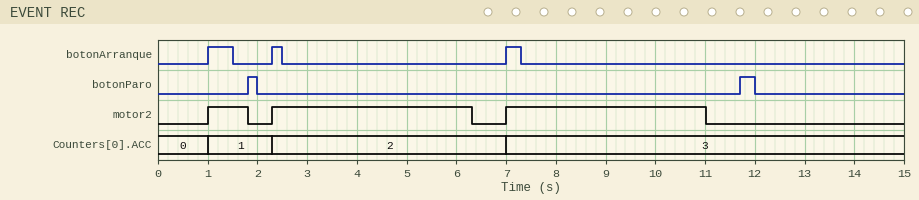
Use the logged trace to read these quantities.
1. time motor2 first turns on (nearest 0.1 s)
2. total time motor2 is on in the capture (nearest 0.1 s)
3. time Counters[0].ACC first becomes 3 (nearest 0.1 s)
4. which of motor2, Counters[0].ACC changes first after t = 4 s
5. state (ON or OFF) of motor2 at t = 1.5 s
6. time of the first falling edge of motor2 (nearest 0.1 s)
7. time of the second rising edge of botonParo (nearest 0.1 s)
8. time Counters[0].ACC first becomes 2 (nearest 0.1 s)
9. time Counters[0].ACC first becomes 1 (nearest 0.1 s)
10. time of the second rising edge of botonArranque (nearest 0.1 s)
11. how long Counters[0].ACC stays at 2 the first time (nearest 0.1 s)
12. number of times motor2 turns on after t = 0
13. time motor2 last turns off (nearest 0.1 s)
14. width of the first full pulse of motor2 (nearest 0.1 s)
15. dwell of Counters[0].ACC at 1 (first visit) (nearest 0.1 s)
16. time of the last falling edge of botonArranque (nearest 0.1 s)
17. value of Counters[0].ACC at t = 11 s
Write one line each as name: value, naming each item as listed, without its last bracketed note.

time motor2 first turns on: 1.0 s
total time motor2 is on in the capture: 8.8 s
time Counters[0].ACC first becomes 3: 7.0 s
which of motor2, Counters[0].ACC changes first after t = 4 s: motor2
state (ON or OFF) of motor2 at t = 1.5 s: ON
time of the first falling edge of motor2: 1.8 s
time of the second rising edge of botonParo: 11.7 s
time Counters[0].ACC first becomes 2: 2.3 s
time Counters[0].ACC first becomes 1: 1.0 s
time of the second rising edge of botonArranque: 2.3 s
how long Counters[0].ACC stays at 2 the first time: 4.7 s
number of times motor2 turns on after t = 0: 3
time motor2 last turns off: 11.0 s
width of the first full pulse of motor2: 0.8 s
dwell of Counters[0].ACC at 1 (first visit): 1.3 s
time of the last falling edge of botonArranque: 7.3 s
value of Counters[0].ACC at t = 11 s: 3
